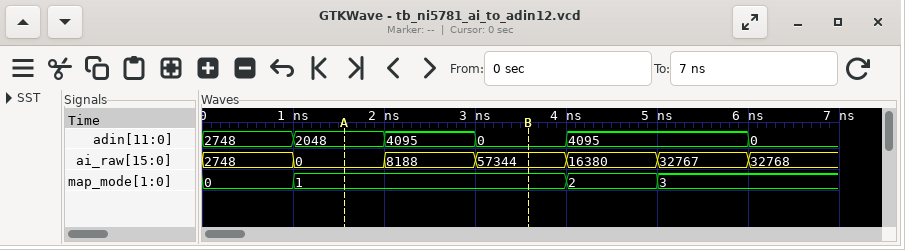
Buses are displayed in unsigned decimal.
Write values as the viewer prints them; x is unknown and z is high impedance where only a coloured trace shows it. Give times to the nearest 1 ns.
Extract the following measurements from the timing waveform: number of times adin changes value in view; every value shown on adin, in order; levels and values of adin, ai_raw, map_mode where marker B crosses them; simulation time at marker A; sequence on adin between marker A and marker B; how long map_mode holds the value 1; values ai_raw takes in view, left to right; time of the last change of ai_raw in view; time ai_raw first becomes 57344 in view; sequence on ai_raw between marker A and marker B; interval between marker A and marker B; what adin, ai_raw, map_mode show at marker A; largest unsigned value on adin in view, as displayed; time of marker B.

5
2748, 2048, 4095, 0, 4095, 0
adin=0, ai_raw=57344, map_mode=1
2 ns
2048, 4095, 0
3 ns
2748, 0, 8188, 57344, 16380, 32767, 32768
6 ns
3 ns
0, 8188, 57344
2 ns
adin=2048, ai_raw=0, map_mode=1
4095
4 ns
